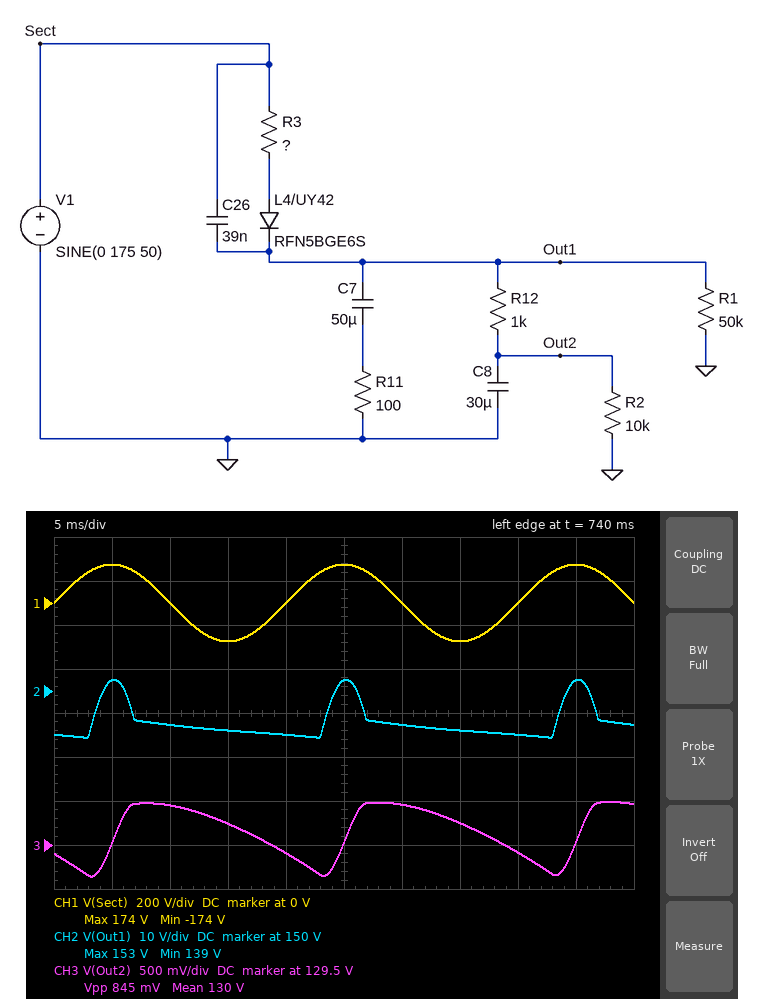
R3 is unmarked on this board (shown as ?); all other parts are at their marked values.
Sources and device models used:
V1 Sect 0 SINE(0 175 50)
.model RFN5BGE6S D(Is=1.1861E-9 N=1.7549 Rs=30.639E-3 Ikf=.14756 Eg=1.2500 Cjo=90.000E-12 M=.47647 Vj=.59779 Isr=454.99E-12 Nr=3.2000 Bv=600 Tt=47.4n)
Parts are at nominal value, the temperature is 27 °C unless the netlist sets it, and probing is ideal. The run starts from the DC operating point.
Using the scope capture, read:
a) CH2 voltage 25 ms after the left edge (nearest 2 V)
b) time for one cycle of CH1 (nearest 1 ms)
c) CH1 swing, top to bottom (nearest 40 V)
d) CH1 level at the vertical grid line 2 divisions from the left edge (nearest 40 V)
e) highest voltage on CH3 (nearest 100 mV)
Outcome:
152 V
20 ms
360 V
0 V
130.0 V
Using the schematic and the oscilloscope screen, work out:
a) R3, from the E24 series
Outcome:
180 Ω
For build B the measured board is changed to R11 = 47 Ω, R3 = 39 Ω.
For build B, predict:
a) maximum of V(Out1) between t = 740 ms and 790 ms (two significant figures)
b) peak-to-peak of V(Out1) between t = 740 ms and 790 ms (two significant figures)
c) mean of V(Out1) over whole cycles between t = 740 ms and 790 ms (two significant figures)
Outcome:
170 V
12 V
160 V
